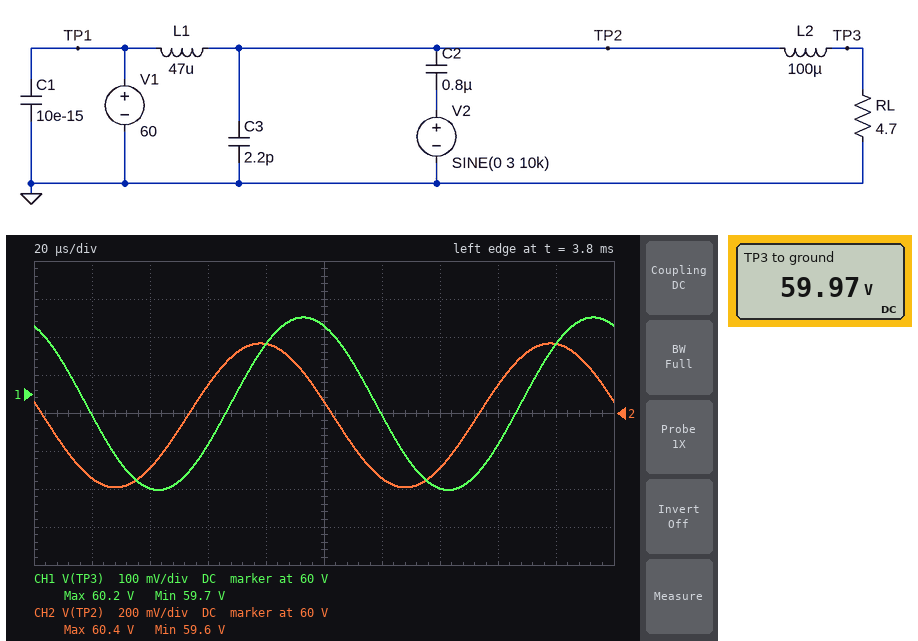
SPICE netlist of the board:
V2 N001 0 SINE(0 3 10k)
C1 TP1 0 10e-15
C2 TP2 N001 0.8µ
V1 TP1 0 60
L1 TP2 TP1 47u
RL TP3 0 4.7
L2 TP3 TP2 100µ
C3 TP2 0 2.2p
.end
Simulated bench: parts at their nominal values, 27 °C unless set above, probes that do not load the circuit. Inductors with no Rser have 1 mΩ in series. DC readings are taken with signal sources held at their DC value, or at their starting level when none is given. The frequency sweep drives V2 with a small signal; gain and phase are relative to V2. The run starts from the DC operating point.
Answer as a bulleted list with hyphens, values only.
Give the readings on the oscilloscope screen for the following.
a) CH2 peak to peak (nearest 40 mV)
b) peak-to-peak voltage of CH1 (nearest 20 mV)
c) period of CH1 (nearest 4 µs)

- 760 mV
- 460 mV
- 100 µs
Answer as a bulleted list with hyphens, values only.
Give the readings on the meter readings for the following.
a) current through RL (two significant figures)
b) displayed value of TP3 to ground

- 13 A
- 59.97 V
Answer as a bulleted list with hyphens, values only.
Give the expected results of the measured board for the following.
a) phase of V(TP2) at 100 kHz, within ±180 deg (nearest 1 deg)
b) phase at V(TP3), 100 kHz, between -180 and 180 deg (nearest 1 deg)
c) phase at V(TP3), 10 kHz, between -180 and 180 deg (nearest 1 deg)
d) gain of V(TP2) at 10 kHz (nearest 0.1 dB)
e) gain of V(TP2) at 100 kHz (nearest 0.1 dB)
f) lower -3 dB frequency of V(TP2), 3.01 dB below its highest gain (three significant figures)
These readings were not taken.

- 0 deg
- -86 deg
- 116 deg
- -18.0 dB
- 0.9 dB
- 30.2 kHz
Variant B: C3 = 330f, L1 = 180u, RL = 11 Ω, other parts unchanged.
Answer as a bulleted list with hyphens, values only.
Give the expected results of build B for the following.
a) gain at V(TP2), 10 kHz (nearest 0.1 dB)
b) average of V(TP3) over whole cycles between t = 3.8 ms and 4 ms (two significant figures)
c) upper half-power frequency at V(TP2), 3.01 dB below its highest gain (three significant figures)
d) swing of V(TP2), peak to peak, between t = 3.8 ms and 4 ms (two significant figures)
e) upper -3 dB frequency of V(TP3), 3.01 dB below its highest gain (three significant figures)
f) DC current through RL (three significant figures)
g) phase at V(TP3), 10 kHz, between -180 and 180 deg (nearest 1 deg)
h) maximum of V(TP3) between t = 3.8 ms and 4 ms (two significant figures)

- -6.3 dB
- 60 V
- 29.7 kHz
- 2.9 V
- 26.4 kHz
- 5.45 A
- 109 deg
- 61 V
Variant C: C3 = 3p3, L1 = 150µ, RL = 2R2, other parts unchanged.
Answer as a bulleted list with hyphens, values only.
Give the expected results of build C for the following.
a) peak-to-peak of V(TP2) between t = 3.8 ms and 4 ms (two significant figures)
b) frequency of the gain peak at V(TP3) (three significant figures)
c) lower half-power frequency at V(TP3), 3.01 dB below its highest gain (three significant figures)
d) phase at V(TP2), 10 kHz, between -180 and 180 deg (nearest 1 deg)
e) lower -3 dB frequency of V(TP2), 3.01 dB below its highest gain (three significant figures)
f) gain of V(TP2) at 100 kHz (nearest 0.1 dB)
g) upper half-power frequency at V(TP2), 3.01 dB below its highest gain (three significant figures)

- 1.5 V
- 22.9 kHz
- 21.9 kHz
- 166 deg
- 22.0 kHz
- 0.5 dB
- 24.1 kHz
